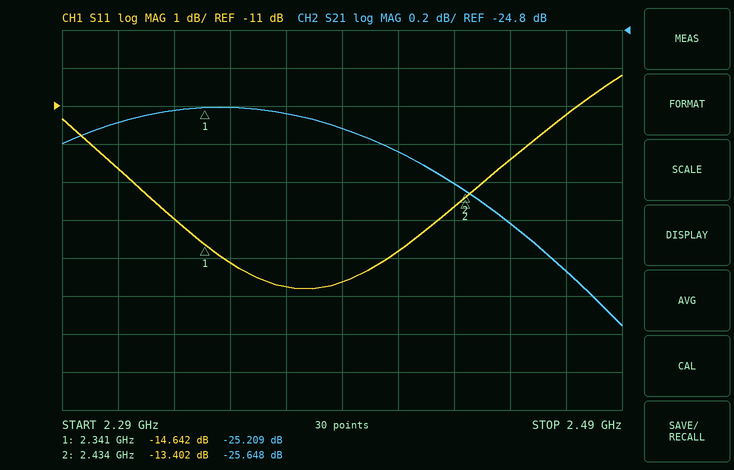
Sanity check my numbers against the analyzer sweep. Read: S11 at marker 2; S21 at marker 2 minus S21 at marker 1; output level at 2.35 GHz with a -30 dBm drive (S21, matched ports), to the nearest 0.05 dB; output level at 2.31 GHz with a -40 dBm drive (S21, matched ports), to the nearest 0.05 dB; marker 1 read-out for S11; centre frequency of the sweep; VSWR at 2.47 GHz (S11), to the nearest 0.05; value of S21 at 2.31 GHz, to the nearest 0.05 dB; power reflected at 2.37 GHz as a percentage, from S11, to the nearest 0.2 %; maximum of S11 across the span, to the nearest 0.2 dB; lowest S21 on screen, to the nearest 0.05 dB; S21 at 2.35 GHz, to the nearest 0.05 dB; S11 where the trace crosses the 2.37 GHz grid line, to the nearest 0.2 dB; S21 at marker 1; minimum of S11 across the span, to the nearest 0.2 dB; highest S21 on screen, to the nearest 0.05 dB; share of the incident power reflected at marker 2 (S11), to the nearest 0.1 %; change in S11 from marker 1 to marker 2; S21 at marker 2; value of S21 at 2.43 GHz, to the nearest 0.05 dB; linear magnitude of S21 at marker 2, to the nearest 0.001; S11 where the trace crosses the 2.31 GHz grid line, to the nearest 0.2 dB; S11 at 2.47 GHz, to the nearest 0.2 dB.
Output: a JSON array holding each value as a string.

["-13.402 dB", "-0.439 dB", "-55.20 dBm", "-65.30 dBm", "-14.642 dB", "2.39 GHz", "1.75", "-25.30 dB", "2.6 %", "-10.2 dB", "-26.35 dB", "-25.20 dB", "-15.8 dB", "-25.209 dB", "-15.8 dB", "-25.20 dB", "4.6 %", "1.240 dB", "-25.648 dB", "-25.60 dB", "0.052", "-12.6 dB", "-11.2 dB"]
